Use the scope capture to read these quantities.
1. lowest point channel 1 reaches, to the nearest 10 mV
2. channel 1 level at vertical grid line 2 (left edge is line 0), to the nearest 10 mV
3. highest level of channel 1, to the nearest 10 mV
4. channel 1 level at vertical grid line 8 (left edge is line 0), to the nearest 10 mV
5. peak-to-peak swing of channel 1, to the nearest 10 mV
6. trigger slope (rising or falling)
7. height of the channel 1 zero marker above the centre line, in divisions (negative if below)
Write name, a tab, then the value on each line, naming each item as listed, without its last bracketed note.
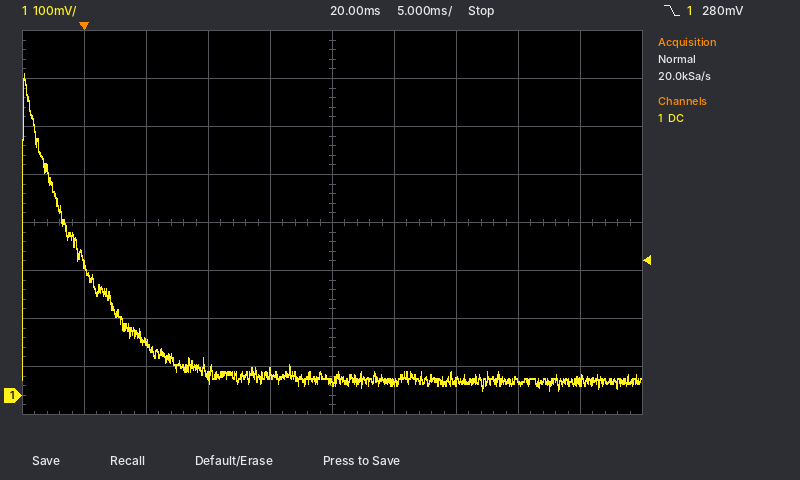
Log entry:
lowest point channel 1 reaches, to the nearest 10 mV	10 mV
channel 1 level at vertical grid line 2 (left edge is line 0), to the nearest 10 mV	110 mV
highest level of channel 1, to the nearest 10 mV	670 mV
channel 1 level at vertical grid line 8 (left edge is line 0), to the nearest 10 mV	30 mV
peak-to-peak swing of channel 1, to the nearest 10 mV	660 mV
trigger slope	falling
height of the channel 1 zero marker above the centre line, in divisions	-3.6 div
